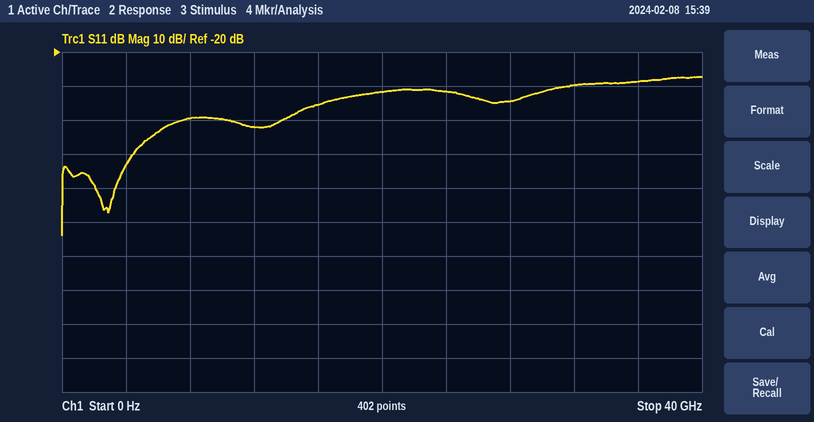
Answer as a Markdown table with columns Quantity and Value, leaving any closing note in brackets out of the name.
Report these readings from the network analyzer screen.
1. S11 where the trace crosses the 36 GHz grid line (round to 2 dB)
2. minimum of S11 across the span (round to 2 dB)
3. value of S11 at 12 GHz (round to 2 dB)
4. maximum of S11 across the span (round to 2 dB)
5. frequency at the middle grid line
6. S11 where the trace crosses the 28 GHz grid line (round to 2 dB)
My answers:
| Quantity | Value |
|---|---|
| S11 where the trace crosses the 36 GHz grid line | -28 dB |
| minimum of S11 across the span | -74 dB |
| value of S11 at 12 GHz | -42 dB |
| maximum of S11 across the span | -28 dB |
| frequency at the middle grid line | 20 GHz |
| S11 where the trace crosses the 28 GHz grid line | -34 dB |
